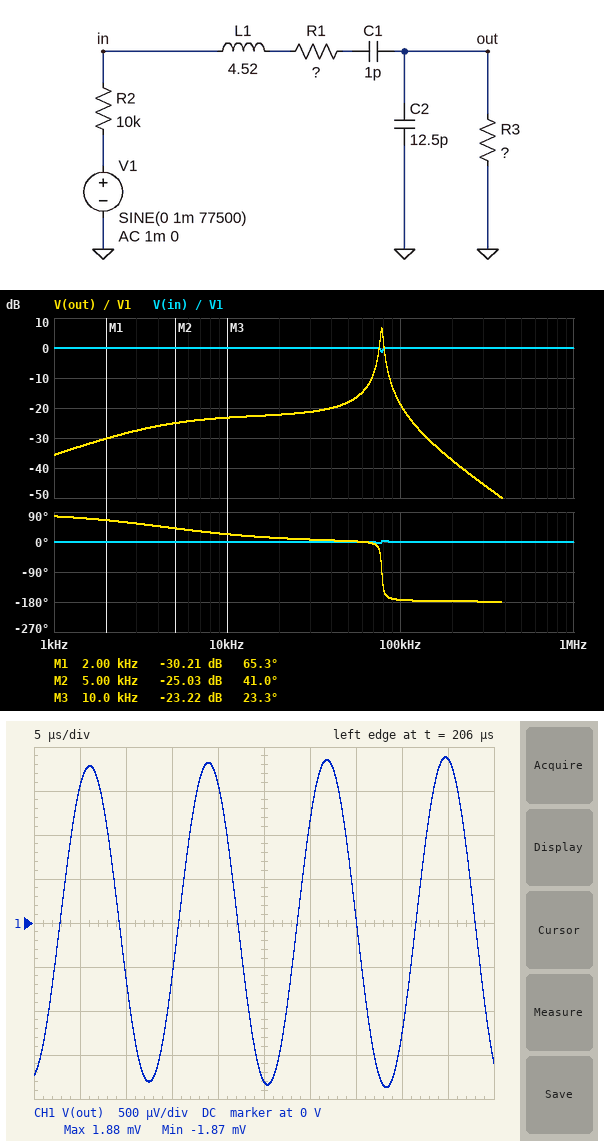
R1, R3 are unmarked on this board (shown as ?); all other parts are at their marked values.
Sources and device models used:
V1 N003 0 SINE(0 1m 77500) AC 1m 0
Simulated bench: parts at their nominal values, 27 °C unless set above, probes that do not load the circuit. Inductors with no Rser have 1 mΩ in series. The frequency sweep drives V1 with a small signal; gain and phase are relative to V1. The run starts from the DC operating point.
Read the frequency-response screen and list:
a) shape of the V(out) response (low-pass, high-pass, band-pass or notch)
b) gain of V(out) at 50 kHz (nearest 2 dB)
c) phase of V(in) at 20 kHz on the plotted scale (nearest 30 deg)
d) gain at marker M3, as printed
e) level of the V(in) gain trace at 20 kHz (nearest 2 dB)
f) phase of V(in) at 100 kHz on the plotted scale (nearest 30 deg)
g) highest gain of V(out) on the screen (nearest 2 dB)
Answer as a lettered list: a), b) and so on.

a) band-pass
b) -18 dB
c) 0 deg
d) -23.22 dB
e) 0 dB
f) 0 deg
g) 6 dB
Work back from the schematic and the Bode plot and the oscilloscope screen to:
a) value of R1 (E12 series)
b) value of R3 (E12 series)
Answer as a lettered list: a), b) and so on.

a) 56 kΩ
b) 2.7 MΩ
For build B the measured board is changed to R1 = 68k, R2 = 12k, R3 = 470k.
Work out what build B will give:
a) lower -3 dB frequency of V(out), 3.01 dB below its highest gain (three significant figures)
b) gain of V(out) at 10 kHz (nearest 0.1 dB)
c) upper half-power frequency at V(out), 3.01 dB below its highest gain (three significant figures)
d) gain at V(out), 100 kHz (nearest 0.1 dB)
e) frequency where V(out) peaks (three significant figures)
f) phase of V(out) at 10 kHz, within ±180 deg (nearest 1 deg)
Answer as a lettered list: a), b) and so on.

a) 75.1 kHz
b) -31.1 dB
c) 79.8 kHz
d) -19.3 dB
e) 77.5 kHz
f) 68 deg
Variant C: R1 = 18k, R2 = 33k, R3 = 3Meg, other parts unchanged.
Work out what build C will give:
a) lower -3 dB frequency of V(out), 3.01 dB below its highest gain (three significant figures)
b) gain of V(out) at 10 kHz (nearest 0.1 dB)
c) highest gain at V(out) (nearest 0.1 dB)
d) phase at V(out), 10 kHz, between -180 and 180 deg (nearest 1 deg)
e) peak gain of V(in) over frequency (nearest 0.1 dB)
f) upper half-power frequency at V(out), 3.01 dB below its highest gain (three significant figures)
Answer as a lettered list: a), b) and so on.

a) 76.7 kHz
b) -23.1 dB
c) 8.7 dB
d) 21 deg
e) 0 dB
f) 78.8 kHz
